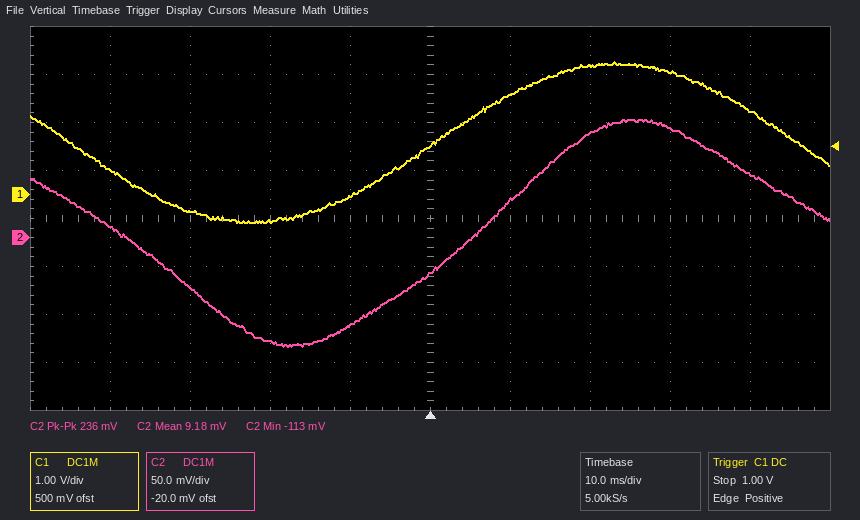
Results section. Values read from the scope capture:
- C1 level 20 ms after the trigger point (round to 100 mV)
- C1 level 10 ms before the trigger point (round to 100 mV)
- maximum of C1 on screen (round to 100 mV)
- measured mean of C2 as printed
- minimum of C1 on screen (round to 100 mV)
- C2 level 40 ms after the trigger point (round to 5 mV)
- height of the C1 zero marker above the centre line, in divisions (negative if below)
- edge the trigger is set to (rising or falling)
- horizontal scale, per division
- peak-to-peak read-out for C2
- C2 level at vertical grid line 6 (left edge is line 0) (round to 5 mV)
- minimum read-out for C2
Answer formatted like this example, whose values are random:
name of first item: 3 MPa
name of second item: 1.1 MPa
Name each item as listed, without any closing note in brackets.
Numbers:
C1 level 20 ms after the trigger point: 2.7 V
C1 level 10 ms before the trigger point: 0.0 V
maximum of C1 on screen: 2.8 V
measured mean of C2 as printed: 9.18 mV
minimum of C1 on screen: -600 mV
C2 level 40 ms after the trigger point: 65 mV
height of the C1 zero marker above the centre line, in divisions: +0.5 div
edge the trigger is set to: rising
horizontal scale, per division: 10 ms
peak-to-peak read-out for C2: 236 mV
C2 level at vertical grid line 6 (left edge is line 0): 40 mV
minimum read-out for C2: -113 mV
